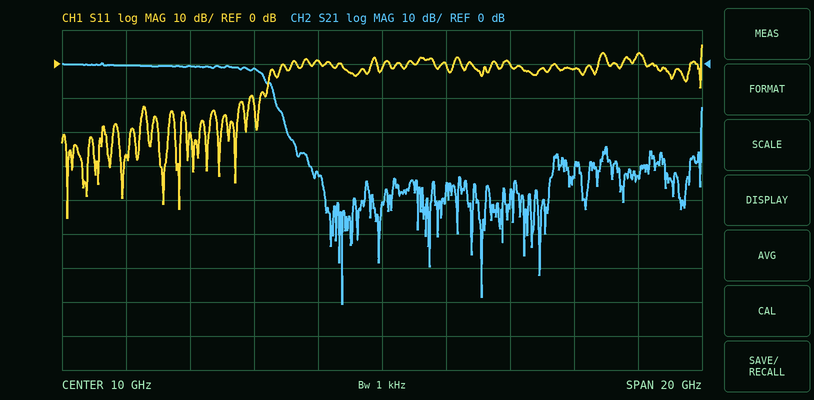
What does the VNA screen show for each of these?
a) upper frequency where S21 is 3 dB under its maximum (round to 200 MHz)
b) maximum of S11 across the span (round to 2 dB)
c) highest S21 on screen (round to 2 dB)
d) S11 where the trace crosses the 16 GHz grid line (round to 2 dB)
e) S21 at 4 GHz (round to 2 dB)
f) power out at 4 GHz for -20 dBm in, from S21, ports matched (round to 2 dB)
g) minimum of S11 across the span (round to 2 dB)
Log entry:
6.2 GHz
6 dB
0 dB
-2 dB
0 dB
-20 dBm
-46 dB
